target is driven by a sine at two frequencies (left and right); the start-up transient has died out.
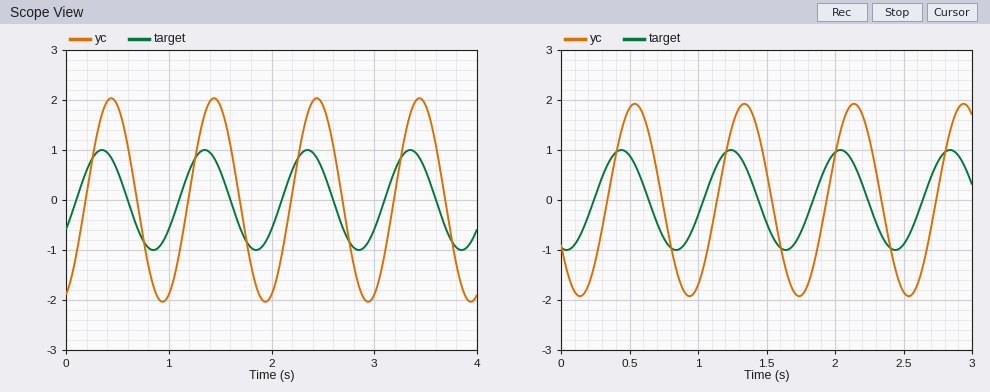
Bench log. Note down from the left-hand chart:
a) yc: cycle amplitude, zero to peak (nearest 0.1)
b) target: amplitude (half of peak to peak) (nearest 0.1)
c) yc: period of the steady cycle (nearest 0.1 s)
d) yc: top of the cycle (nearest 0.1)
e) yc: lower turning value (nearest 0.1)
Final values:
2.0
1.0
1.0 s
2.0
-2.0
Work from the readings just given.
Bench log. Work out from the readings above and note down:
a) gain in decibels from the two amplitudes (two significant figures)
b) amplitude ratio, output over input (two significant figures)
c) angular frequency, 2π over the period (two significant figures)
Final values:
6.0 dB
2.0
6.3 rad/s
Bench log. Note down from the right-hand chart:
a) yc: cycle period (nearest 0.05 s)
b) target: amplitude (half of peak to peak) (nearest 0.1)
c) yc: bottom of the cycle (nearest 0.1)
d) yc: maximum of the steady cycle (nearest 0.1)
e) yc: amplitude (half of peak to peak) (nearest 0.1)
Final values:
0.80 s
1.0
-1.9
1.9
1.9
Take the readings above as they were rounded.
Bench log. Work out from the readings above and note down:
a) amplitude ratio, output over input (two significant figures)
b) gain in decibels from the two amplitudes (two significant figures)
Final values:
1.9
5.6 dB
